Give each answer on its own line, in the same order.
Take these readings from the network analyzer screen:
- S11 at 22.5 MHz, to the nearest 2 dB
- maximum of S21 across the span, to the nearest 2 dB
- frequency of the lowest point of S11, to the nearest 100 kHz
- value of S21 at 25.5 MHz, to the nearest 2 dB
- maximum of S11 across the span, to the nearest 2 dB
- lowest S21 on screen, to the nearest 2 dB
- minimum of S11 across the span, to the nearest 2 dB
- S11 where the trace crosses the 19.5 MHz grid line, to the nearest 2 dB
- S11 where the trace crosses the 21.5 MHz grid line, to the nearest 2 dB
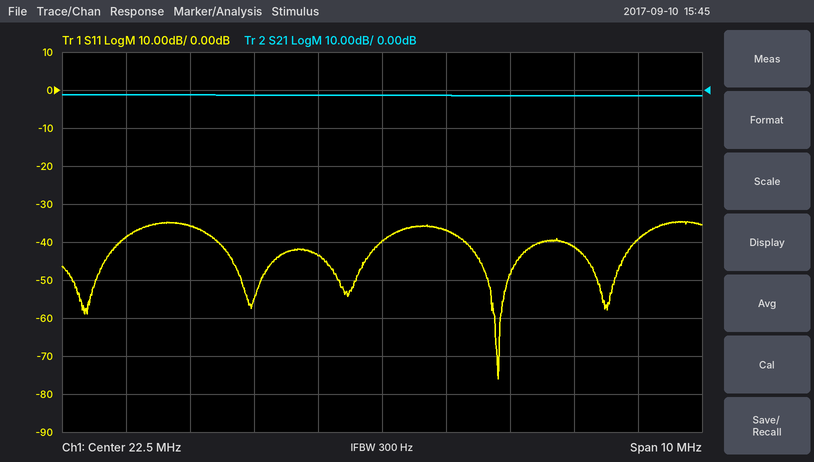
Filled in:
-40 dB
-2 dB
24.3 MHz
-2 dB
-34 dB
-2 dB
-76 dB
-36 dB
-44 dB
